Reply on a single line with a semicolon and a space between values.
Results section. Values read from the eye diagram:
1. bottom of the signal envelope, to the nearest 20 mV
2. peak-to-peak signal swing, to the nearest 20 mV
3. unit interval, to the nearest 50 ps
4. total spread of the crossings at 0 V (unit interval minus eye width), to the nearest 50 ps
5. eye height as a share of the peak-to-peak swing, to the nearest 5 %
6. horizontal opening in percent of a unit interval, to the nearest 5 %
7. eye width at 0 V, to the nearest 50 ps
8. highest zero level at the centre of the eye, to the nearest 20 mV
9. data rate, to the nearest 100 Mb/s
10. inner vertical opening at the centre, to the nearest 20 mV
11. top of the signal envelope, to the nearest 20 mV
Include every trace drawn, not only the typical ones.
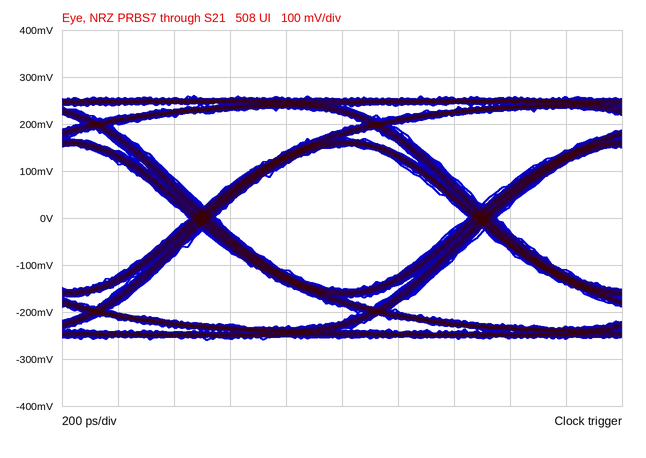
-260 mV; 520 mV; 1.00 ns; 100 ps; 60 %; 90 %; 900 ps; -160 mV; 1.0 Gb/s; 300 mV; 260 mV
